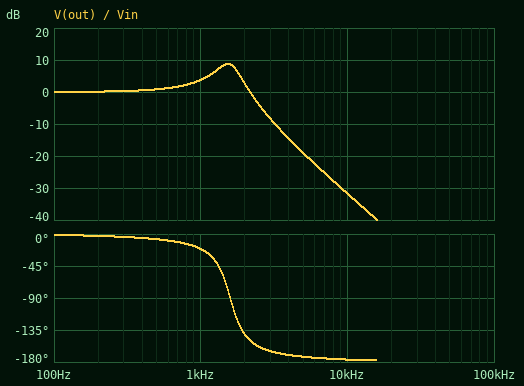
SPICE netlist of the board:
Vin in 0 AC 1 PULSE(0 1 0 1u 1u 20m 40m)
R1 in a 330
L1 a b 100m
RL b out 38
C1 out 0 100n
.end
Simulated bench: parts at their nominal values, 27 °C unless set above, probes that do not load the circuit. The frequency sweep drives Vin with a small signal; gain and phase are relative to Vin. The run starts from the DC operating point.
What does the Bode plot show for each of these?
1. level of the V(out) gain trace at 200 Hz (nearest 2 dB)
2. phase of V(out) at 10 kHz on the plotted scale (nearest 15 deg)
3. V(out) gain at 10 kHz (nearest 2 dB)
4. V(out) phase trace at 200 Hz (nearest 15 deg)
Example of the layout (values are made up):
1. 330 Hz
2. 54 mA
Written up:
1. 0 dB
2. -180 deg
3. -32 dB
4. 0 deg
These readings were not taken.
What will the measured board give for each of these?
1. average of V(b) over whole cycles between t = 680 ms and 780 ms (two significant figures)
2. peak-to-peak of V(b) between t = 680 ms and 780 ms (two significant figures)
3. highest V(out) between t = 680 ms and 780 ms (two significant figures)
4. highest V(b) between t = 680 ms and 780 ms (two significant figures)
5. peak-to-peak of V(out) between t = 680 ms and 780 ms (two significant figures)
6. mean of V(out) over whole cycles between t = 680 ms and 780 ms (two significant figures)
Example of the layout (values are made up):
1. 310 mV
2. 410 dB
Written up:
1. 500 mV
2. 2.1 V
3. 1.6 V
4. 1.6 V
5. 2.1 V
6. 500 mV
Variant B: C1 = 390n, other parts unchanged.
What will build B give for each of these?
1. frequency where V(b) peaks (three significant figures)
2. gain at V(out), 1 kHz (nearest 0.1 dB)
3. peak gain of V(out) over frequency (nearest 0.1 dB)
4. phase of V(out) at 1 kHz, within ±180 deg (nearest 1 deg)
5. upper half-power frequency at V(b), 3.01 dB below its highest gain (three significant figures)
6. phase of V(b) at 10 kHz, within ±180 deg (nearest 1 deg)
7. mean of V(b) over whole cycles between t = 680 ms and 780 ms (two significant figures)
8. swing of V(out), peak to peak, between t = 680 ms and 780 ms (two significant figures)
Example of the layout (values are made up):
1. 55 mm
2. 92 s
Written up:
1. 692 Hz
2. -0.4 dB
3. 3.4 dB
4. -121 deg
5. 959 Hz
6. -134 deg
7. 500 mV
8. 1.6 V
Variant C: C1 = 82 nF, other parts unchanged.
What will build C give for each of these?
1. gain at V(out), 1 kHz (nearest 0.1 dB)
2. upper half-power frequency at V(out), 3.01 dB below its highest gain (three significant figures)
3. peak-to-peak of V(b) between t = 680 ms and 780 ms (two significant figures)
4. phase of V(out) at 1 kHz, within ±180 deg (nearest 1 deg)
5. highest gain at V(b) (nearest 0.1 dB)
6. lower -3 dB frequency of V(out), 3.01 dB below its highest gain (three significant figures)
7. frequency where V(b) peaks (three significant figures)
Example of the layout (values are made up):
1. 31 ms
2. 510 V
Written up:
1. 3.1 dB
2. 1.98 kHz
3. 2.2 V
4. -16 deg
5. 9.7 dB
6. 1.38 kHz
7. 1.71 kHz
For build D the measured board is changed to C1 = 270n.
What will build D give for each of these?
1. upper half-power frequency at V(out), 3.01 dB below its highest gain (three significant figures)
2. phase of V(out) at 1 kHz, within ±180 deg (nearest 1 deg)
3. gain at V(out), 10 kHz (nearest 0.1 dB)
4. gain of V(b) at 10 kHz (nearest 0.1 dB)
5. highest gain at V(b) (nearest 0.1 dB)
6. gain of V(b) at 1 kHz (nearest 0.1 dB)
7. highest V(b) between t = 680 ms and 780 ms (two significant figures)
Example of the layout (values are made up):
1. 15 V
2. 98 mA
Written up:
1. 1.14 kHz
2. -96 deg
3. -40.5 dB
4. -39.0 dB
5. 4.8 dB
6. 4.1 dB
7. 1.4 V
